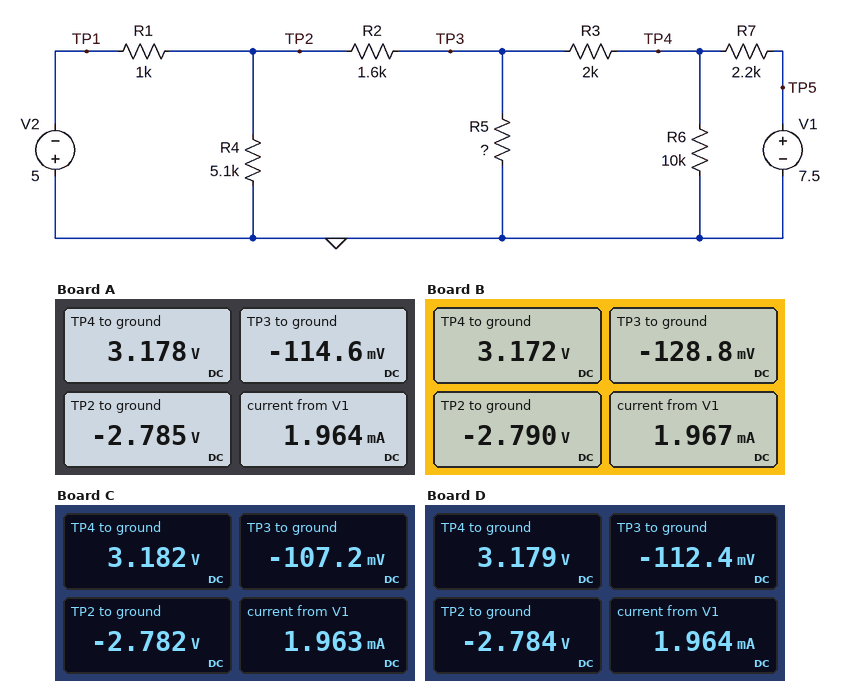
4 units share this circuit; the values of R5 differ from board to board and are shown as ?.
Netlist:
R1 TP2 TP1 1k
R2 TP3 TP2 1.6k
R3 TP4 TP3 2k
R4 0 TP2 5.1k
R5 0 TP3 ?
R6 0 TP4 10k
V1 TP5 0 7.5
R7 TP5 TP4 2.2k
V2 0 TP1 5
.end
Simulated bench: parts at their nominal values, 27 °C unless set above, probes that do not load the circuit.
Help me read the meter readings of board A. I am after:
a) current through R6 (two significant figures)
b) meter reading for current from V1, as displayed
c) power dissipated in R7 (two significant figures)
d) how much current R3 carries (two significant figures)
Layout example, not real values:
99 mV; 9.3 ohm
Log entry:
320 µA; 1.964 mA; 8.5 mW; 1.6 mA
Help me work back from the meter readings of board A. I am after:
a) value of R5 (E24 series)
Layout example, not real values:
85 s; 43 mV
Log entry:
5.1 kΩ
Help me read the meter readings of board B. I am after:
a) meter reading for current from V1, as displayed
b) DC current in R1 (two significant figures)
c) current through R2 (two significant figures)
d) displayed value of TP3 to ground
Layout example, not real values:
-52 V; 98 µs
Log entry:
1.967 mA; 2.2 mA; 1.7 mA; -128.8 mV
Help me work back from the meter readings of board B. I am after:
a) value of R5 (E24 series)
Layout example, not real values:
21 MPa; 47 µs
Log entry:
10 kΩ
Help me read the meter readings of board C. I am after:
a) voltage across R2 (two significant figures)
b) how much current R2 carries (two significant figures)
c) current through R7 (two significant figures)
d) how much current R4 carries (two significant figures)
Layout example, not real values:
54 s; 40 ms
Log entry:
2.7 V; 1.7 mA; 2.0 mA; 550 µA
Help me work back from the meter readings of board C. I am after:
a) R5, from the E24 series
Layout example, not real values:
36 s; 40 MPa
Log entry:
3.9 kΩ
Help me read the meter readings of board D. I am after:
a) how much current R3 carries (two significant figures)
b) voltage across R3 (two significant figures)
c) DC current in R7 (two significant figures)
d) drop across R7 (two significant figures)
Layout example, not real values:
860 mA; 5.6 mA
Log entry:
1.6 mA; 3.3 V; 2.0 mA; 4.3 V
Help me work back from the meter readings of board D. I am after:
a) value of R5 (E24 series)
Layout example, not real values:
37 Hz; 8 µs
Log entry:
4.7 kΩ
